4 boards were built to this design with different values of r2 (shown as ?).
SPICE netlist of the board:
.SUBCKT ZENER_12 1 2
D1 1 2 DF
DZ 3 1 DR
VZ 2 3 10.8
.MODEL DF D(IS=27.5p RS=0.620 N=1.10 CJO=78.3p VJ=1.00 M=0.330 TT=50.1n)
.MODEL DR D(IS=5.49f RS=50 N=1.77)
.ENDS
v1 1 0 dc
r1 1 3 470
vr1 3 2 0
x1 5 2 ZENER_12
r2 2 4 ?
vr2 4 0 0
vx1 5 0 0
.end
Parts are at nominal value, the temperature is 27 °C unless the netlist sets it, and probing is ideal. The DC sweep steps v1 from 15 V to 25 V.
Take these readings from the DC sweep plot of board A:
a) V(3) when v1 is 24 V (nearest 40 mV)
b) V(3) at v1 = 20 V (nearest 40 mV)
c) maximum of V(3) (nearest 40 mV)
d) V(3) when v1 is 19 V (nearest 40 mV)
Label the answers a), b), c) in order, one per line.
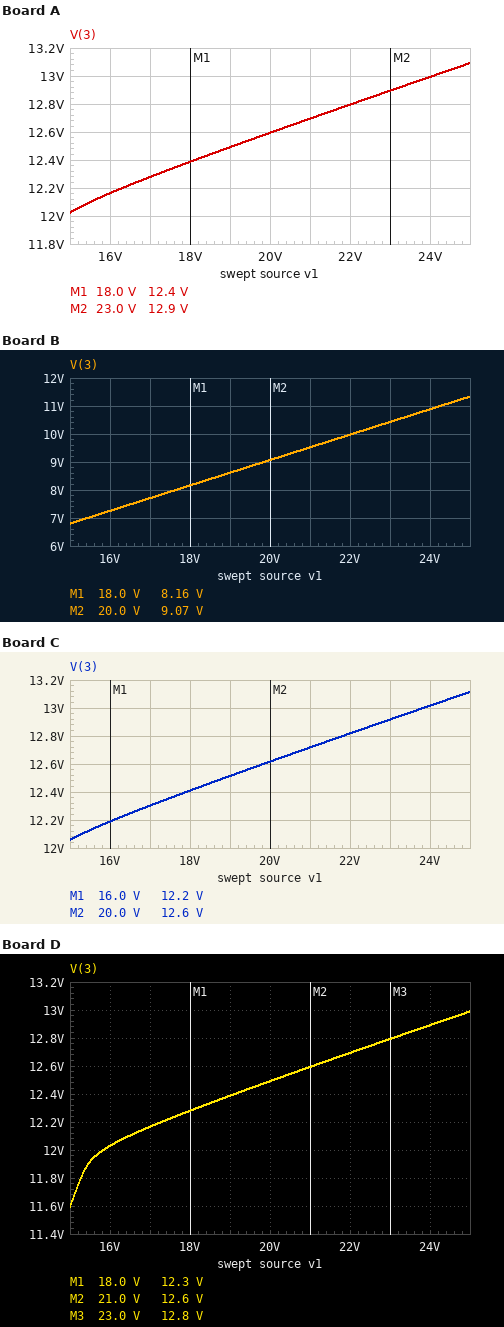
a) 13.00 V
b) 12.60 V
c) 13.08 V
d) 12.48 V
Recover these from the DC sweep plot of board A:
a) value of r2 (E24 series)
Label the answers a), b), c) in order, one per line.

a) 2.2 kΩ
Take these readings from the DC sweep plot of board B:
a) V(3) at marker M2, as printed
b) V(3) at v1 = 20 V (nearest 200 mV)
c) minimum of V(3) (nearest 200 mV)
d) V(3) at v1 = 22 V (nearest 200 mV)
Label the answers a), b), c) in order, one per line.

a) 9.07 V
b) 9.0 V
c) 6.8 V
d) 10.0 V
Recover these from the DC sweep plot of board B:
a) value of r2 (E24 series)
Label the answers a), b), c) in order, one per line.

a) 390 Ω
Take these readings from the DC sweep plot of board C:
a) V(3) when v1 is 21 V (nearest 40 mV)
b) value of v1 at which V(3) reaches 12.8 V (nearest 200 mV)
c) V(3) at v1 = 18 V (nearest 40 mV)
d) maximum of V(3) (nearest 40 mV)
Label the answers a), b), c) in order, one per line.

a) 12.72 V
b) 21.8 V
c) 12.40 V
d) 13.12 V
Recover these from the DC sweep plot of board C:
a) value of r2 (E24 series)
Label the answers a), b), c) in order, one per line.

a) 2.4 kΩ
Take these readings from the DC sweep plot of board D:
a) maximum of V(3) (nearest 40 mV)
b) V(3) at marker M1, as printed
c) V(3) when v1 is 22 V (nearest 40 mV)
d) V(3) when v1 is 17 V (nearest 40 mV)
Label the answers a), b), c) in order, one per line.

a) 13.00 V
b) 12.3 V
c) 12.68 V
d) 12.16 V
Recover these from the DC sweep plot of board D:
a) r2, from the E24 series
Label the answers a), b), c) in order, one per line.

a) 1.6 kΩ
